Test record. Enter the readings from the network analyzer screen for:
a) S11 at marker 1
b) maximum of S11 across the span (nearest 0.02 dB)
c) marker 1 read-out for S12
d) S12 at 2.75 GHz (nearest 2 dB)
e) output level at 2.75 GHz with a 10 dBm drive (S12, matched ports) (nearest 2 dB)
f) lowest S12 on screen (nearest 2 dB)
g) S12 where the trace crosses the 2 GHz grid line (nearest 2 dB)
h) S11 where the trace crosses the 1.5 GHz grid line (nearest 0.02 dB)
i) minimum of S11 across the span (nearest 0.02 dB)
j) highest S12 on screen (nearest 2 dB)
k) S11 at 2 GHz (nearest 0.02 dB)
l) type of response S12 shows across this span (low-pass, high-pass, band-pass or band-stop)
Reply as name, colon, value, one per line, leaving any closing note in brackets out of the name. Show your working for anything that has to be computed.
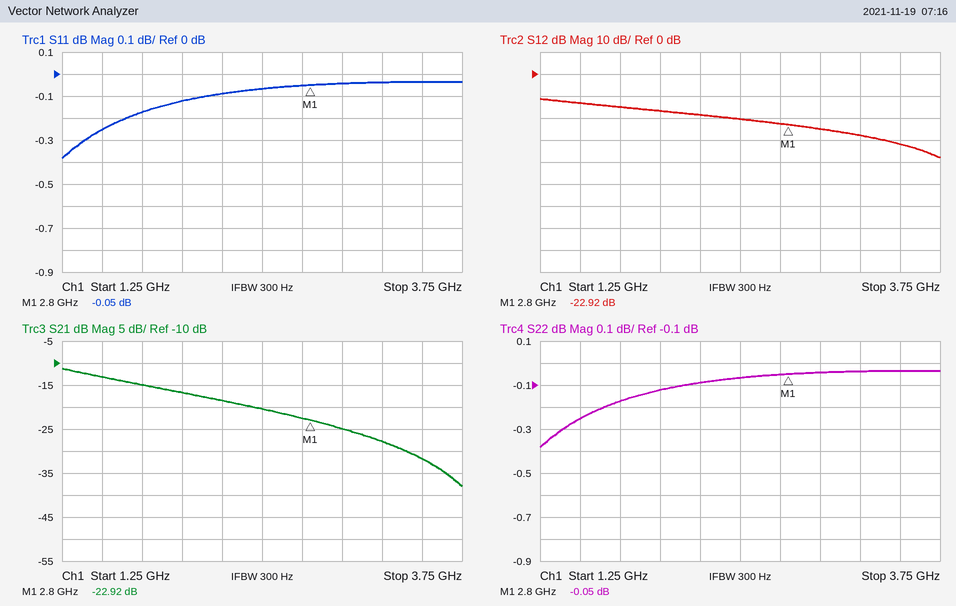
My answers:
S11 at marker 1: -0.05 dB
maximum of S11 across the span: -0.04 dB
marker 1 read-out for S12: -22.92 dB
S12 at 2.75 GHz: -22 dB
output level at 2.75 GHz with a 10 dBm drive (S12, matched ports): 10 dBm + (-22 dB) = -12 dBm
lowest S12 on screen: -38 dB
S12 where the trace crosses the 2 GHz grid line: -16 dB
S11 where the trace crosses the 1.5 GHz grid line: -0.26 dB
minimum of S11 across the span: -0.38 dB
highest S12 on screen: -12 dB
S11 at 2 GHz: -0.12 dB
type of response S12 shows across this span: low-pass
